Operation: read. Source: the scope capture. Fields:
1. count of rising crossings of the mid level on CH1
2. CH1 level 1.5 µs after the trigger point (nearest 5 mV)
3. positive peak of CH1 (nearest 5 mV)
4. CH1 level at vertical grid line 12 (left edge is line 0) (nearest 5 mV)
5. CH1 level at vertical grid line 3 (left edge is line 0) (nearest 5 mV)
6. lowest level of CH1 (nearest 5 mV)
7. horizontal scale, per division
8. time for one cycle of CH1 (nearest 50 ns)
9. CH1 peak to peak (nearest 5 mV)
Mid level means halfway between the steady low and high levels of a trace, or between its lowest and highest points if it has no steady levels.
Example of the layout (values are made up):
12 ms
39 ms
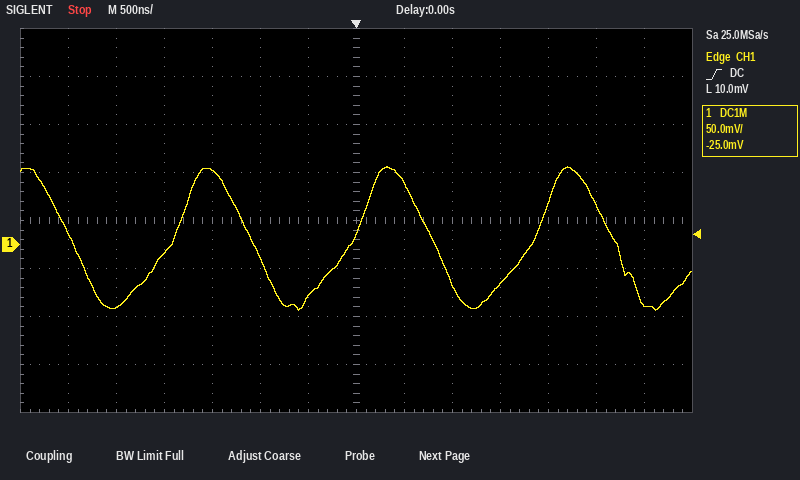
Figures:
3
-40 mV
80 mV
40 mV
-10 mV
-70 mV
500 ns
1.90 µs
150 mV
